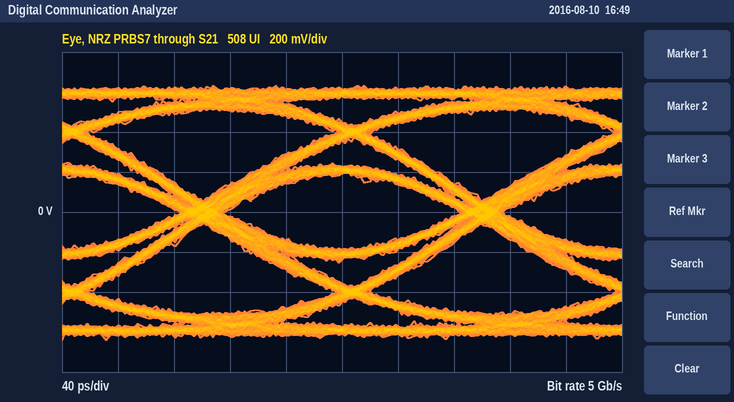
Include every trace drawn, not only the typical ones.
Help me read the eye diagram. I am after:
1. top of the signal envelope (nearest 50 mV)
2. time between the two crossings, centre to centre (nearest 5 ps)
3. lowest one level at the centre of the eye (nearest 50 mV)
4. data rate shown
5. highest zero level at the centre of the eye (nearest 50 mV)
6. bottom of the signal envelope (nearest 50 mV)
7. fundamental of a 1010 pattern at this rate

650 mV
200 ps
200 mV
5 Gb/s
-200 mV
-650 mV
2.5 GHz
